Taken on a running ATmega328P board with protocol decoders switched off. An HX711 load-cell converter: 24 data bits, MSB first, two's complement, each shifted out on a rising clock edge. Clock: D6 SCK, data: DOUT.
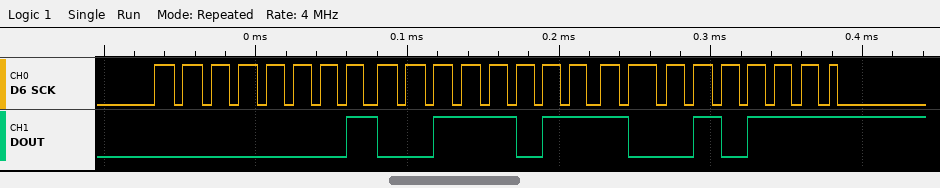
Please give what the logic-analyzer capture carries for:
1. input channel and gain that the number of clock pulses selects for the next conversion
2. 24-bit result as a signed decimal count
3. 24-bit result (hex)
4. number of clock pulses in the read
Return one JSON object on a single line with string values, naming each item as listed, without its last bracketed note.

{"input channel and gain that the number of clock pulses selects for the next conversion": "channel A, gain 128", "24-bit result as a signed decimal count": "80791", "24-bit result": "0x013B97", "number of clock pulses in the read": "25"}
